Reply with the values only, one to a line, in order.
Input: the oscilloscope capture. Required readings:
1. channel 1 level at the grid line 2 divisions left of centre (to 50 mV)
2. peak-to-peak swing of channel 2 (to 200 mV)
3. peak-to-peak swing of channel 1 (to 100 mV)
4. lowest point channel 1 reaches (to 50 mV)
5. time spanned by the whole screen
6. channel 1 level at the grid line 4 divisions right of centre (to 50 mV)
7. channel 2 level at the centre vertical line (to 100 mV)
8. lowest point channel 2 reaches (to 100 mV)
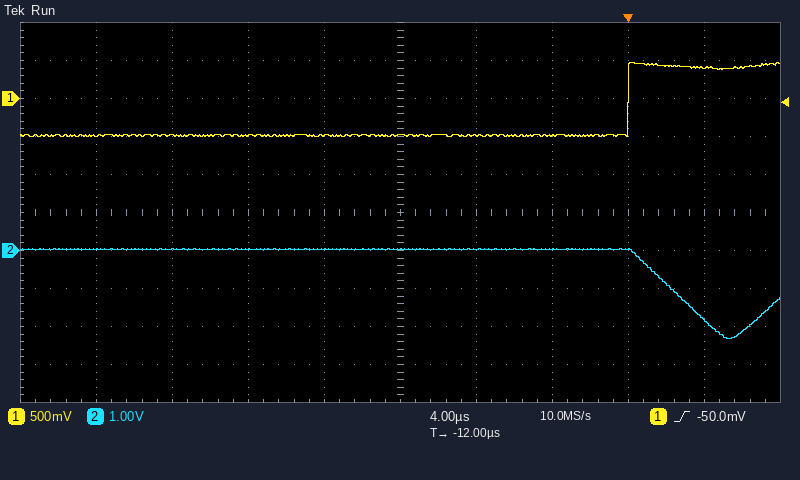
-500 mV
2.4 V
1.00 V
-500 mV
40 µs
400 mV
0.0 V
-2.3 V
